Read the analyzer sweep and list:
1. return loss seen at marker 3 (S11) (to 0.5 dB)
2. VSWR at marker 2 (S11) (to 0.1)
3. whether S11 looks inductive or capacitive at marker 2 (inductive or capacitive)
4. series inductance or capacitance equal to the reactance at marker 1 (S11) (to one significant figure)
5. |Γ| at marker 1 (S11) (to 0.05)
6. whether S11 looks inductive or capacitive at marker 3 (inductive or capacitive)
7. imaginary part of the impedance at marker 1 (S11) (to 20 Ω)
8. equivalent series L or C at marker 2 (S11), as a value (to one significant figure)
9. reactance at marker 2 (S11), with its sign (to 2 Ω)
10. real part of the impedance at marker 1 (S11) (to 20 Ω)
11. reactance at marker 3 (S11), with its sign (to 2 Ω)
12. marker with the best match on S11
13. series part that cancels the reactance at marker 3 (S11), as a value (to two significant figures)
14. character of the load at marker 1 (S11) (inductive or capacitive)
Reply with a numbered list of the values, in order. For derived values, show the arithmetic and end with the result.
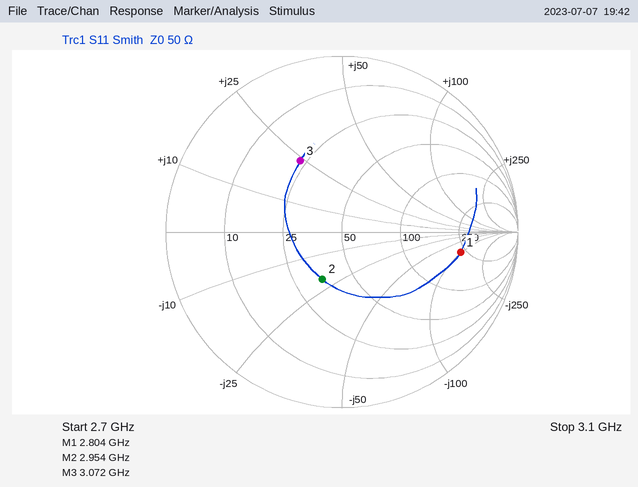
1. 6.5 dB
2. 1.8
3. capacitive
4. C = 1/(2π × 2.804 GHz × 100 Ω) ≈ 568 fF, so 600 fF to one significant figure
5. 0.70
6. inductive
7. -100 Ω
8. C = 1/(2π × 2.954 GHz × 20 Ω) ≈ 3 pF
9. -20 Ω
10. 220 Ω
11. +24 Ω
12. marker 2
13. C = 1/(2π × 3.072 GHz × 24 Ω) ≈ 2.2 pF
14. capacitive
